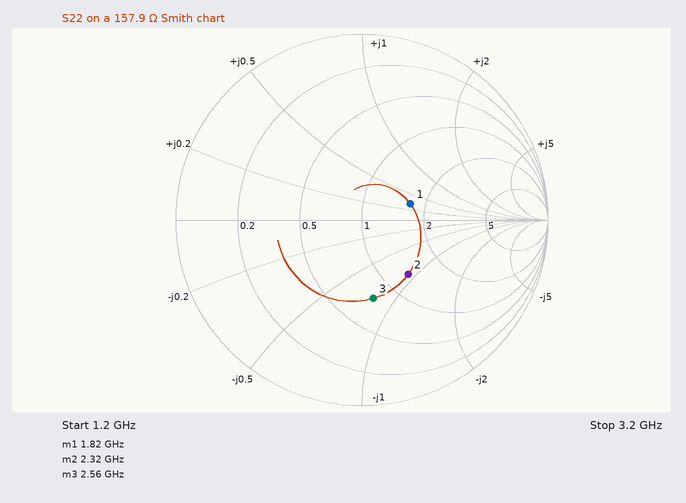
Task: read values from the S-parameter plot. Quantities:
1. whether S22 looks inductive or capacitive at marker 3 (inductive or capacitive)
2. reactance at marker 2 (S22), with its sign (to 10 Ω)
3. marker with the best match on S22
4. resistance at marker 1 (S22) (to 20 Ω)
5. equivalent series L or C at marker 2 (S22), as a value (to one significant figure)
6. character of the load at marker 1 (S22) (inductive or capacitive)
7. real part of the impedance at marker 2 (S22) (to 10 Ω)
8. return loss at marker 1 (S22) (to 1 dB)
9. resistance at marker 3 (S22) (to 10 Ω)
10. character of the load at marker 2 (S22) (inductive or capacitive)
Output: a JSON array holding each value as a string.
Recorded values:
["capacitive", "-140 Ω", "marker 1", "260 Ω", "500 fF", "inductive", "210 Ω", "11 dB", "120 Ω", "capacitive"]
